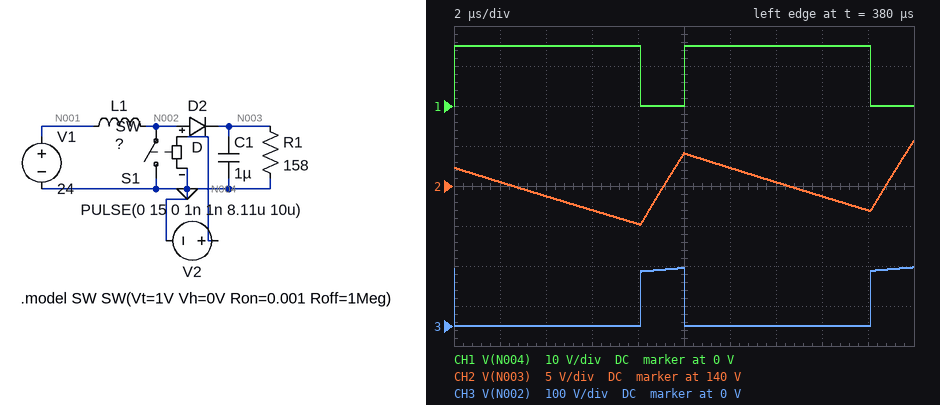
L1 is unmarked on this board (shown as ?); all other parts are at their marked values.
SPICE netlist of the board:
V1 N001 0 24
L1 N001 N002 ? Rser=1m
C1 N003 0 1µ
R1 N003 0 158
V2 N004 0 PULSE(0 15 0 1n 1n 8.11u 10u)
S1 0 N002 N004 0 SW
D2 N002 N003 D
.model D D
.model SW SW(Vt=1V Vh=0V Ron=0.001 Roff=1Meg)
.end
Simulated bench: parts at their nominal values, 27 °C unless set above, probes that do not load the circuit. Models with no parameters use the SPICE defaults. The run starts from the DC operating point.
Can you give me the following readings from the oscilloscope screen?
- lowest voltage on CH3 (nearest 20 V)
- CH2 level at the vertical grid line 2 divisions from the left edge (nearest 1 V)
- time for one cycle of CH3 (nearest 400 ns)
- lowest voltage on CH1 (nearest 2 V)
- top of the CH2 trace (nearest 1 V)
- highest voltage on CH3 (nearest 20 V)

0 V
139 V
10.0 µs
0 V
146 V
140 V
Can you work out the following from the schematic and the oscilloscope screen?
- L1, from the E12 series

680 µH
